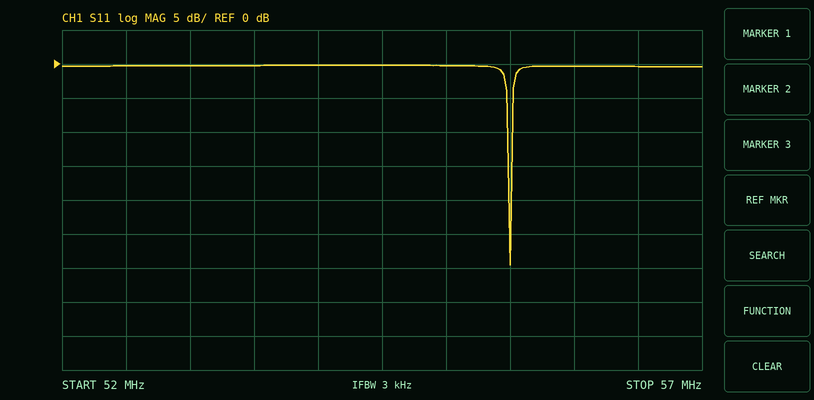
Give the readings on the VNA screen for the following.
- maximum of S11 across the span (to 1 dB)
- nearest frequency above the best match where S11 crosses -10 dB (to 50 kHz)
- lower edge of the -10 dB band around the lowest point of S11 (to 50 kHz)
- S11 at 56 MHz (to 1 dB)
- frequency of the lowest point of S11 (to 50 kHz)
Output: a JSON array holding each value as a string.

["0 dB", "55.50 MHz", "55.50 MHz", "0 dB", "55.50 MHz"]
